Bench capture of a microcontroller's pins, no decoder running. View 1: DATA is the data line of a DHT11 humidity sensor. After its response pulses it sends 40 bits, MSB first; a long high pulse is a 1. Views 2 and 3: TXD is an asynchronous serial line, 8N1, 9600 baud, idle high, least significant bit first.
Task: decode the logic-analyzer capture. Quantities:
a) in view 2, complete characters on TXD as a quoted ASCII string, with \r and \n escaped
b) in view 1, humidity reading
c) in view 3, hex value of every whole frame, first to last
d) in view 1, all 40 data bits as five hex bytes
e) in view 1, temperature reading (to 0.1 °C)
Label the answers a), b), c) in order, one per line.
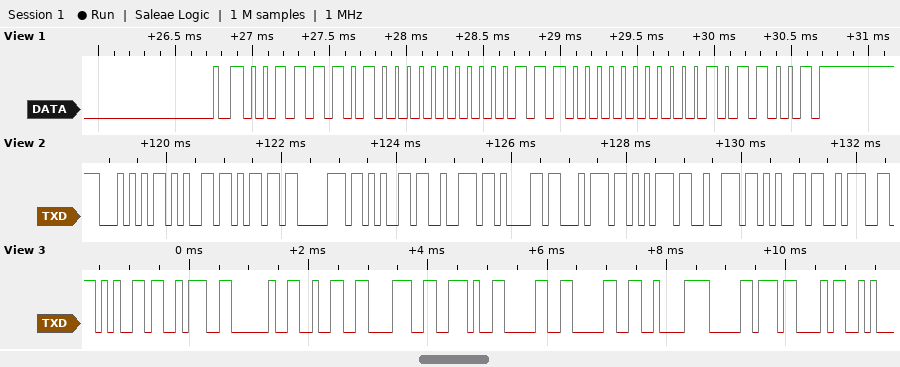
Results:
a) "Temperature:"
b) 61 %
c) 65 3A 20 32 38 2E 30 30 C2 B0 43
d) 3D 00 1C 00 59
e) 28.0 °C
